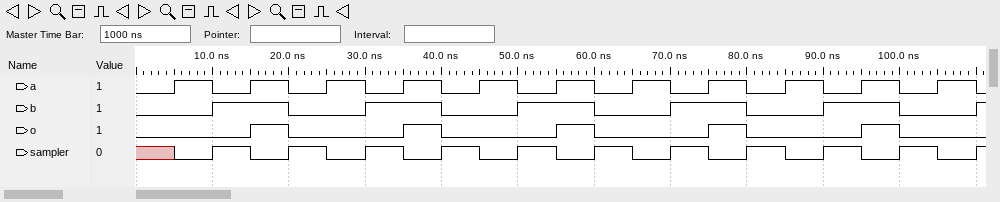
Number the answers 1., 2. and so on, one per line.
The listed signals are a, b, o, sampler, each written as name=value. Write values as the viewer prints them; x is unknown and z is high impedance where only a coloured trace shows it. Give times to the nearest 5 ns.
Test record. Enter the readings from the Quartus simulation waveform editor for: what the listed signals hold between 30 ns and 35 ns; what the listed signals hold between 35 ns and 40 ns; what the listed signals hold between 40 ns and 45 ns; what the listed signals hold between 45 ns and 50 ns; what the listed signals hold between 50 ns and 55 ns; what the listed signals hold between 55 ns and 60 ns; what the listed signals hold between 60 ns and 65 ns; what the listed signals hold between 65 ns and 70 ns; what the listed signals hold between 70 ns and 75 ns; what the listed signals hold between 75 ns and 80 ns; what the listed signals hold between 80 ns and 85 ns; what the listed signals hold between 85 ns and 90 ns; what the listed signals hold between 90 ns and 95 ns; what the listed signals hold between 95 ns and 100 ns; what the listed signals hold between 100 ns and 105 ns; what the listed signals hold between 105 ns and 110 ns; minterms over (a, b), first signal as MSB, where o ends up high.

1. a=0, b=1, o=0, sampler=1
2. a=1, b=1, o=1, sampler=0
3. a=0, b=0, o=0, sampler=1
4. a=1, b=0, o=0, sampler=0
5. a=0, b=1, o=0, sampler=1
6. a=1, b=1, o=1, sampler=0
7. a=0, b=0, o=0, sampler=1
8. a=1, b=0, o=0, sampler=0
9. a=0, b=1, o=0, sampler=1
10. a=1, b=1, o=1, sampler=0
11. a=0, b=0, o=0, sampler=1
12. a=1, b=0, o=0, sampler=0
13. a=0, b=1, o=0, sampler=1
14. a=1, b=1, o=1, sampler=0
15. a=0, b=0, o=0, sampler=1
16. a=1, b=0, o=0, sampler=0
17. 3
